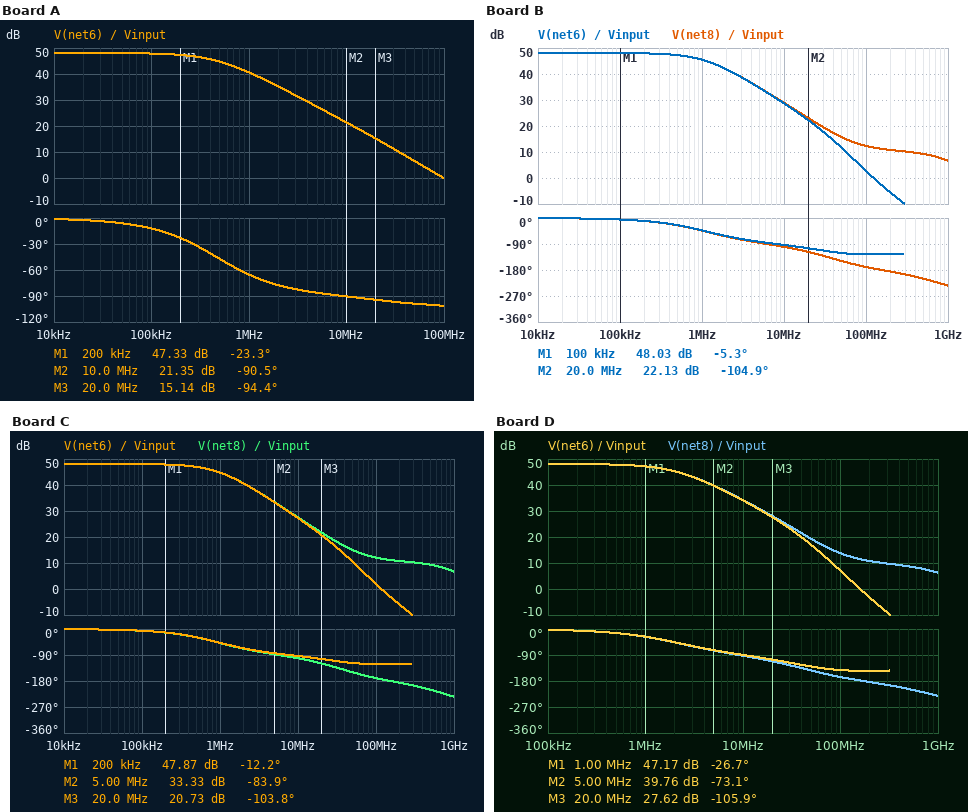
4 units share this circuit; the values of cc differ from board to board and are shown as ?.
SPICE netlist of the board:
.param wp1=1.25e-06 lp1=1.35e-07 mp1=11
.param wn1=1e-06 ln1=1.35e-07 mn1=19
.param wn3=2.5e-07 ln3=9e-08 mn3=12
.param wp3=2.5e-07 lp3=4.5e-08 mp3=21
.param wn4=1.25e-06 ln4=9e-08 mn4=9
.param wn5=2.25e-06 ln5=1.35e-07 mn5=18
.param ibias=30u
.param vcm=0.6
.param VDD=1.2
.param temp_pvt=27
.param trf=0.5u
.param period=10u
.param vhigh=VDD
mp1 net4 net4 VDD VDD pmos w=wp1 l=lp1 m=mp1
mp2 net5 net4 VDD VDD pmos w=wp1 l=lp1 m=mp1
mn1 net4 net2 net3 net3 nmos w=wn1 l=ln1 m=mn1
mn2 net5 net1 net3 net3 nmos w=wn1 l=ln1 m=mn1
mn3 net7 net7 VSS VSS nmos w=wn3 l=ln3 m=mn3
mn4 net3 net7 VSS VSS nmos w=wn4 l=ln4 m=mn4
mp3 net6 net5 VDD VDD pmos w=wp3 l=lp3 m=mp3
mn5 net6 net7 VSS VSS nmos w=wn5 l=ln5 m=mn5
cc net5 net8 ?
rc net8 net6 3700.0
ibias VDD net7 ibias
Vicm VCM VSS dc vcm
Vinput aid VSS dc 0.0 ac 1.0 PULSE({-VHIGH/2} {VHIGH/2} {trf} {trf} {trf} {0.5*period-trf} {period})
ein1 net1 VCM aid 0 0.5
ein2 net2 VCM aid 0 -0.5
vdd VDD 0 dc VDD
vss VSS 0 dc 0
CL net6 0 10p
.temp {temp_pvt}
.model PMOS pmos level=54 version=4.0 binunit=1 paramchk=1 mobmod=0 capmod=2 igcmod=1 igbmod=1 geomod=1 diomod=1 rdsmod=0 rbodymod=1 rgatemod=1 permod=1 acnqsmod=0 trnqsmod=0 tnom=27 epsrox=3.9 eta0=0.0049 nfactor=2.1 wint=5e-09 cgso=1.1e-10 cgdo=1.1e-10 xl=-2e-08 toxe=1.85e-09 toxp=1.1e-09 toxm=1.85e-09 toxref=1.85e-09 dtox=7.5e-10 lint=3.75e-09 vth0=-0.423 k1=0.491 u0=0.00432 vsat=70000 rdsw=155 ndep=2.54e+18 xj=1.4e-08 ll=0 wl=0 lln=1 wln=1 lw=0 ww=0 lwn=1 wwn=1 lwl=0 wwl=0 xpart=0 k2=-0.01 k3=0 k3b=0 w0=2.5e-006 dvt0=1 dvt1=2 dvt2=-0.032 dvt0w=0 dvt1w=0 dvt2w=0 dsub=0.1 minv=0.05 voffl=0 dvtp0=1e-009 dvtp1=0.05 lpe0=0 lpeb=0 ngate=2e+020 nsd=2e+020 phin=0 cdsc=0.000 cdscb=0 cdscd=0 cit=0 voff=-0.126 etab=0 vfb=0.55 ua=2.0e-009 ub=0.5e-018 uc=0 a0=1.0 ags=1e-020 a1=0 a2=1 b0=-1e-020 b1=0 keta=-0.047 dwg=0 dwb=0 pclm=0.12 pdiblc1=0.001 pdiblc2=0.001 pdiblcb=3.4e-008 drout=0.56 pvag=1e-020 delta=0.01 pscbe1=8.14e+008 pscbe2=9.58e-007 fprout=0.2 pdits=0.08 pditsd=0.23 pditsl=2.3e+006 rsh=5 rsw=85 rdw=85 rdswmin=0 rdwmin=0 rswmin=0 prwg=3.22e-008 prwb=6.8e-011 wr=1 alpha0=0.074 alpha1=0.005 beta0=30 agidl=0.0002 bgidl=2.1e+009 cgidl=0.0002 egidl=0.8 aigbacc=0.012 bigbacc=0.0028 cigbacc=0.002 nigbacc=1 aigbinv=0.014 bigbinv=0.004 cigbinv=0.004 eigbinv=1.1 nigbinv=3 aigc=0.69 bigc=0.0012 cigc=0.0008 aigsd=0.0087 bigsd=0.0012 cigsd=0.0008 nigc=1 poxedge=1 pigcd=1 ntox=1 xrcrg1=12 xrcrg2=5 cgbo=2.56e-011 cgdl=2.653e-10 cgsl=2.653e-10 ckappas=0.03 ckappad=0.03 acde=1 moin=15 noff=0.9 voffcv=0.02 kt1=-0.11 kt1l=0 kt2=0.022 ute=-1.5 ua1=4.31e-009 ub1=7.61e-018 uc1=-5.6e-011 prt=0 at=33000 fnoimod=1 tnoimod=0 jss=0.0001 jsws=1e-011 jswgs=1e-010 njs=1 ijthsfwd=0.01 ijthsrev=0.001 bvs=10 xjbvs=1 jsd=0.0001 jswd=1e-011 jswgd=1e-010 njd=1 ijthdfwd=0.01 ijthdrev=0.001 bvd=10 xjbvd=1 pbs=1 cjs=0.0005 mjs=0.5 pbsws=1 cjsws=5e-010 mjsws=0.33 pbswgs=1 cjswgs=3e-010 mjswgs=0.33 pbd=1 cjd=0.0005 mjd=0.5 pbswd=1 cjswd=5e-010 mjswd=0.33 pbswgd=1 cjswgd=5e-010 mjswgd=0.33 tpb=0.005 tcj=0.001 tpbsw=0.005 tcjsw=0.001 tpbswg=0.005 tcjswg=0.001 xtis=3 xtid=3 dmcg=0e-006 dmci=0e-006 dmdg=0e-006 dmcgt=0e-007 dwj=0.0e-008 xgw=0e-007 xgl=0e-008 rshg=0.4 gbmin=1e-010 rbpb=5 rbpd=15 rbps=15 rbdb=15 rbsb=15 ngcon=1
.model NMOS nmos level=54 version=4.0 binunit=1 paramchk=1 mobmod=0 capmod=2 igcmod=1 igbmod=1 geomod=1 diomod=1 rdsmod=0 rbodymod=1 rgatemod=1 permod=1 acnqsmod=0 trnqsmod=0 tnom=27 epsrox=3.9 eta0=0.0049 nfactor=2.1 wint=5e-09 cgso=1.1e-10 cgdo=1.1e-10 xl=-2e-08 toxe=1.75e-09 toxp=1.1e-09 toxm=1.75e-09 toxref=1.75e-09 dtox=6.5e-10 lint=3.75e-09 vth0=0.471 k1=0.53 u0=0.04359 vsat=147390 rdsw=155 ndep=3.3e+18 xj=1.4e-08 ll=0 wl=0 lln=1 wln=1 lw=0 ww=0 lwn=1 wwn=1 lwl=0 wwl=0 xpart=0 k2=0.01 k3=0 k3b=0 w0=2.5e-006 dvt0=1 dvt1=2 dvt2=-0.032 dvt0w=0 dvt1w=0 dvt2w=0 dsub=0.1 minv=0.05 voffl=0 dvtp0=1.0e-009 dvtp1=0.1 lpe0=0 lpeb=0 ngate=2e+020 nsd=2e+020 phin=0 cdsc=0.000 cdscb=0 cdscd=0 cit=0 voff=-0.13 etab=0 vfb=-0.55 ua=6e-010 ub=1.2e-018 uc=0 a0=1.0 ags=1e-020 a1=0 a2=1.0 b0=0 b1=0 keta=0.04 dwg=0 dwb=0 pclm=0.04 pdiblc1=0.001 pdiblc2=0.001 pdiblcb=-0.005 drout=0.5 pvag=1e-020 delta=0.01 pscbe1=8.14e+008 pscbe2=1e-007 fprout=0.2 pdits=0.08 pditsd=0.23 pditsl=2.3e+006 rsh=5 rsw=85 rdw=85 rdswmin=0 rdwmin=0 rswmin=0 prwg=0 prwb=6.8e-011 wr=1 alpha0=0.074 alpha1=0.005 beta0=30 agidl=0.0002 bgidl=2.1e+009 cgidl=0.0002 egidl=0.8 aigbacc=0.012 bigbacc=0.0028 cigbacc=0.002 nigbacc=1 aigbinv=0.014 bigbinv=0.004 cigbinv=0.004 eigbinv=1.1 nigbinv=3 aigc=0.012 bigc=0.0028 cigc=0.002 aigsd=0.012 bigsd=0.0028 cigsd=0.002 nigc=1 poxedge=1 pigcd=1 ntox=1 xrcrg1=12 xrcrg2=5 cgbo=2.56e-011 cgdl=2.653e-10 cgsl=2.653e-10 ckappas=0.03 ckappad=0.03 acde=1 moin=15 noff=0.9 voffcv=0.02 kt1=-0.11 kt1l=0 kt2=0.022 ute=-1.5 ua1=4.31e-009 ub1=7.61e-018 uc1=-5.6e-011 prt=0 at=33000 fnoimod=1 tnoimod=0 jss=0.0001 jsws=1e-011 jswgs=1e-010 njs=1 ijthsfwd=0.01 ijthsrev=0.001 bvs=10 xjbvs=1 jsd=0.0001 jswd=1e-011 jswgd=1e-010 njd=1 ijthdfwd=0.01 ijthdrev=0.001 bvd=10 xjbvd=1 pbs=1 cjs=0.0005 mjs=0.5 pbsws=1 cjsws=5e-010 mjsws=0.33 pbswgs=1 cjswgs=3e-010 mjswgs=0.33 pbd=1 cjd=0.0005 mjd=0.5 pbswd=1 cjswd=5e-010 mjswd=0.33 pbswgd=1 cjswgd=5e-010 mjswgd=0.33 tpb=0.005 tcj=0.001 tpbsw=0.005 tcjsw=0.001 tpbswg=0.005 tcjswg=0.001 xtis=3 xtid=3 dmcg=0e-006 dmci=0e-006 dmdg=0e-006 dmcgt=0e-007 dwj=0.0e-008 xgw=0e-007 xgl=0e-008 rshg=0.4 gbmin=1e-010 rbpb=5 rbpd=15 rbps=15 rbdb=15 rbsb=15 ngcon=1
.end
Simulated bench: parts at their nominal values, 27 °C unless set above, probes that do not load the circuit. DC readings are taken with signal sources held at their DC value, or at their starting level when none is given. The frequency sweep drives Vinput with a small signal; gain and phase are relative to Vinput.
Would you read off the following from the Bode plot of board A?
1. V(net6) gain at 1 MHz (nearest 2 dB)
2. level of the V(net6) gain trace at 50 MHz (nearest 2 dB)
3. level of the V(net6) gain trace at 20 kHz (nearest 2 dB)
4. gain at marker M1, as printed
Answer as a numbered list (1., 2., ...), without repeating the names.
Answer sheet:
1. 40 dB
2. 6 dB
3. 48 dB
4. 47.33 dB
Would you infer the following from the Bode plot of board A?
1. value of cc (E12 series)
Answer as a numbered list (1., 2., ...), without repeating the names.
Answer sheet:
1. 1 pF
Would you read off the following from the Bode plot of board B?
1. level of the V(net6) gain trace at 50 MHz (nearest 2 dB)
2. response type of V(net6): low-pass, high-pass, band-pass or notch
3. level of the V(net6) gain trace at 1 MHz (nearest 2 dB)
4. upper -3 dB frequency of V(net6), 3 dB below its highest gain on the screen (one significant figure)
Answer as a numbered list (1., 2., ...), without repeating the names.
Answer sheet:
1. 12 dB
2. low-pass
3. 46 dB
4. 1 MHz
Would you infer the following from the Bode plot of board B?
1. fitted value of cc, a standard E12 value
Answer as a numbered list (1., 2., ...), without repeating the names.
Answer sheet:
1. 390 fF
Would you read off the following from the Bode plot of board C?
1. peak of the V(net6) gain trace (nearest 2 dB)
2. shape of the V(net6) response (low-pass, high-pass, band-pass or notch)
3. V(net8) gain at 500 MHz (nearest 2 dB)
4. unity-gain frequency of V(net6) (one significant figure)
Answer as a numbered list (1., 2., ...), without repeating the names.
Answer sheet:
1. 48 dB
2. low-pass
3. 10 dB
4. 100 MHz
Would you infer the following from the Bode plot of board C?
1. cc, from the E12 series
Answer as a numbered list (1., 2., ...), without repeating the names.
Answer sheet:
1. 470 fF
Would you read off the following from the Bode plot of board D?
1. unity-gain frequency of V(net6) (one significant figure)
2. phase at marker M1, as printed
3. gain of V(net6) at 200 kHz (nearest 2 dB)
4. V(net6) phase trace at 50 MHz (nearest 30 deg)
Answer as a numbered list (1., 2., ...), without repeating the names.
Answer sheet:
1. 200 MHz
2. -26.7 deg
3. 48 dB
4. -120 deg
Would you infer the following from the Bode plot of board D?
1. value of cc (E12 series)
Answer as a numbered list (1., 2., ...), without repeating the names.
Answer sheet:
1. 180 fF
